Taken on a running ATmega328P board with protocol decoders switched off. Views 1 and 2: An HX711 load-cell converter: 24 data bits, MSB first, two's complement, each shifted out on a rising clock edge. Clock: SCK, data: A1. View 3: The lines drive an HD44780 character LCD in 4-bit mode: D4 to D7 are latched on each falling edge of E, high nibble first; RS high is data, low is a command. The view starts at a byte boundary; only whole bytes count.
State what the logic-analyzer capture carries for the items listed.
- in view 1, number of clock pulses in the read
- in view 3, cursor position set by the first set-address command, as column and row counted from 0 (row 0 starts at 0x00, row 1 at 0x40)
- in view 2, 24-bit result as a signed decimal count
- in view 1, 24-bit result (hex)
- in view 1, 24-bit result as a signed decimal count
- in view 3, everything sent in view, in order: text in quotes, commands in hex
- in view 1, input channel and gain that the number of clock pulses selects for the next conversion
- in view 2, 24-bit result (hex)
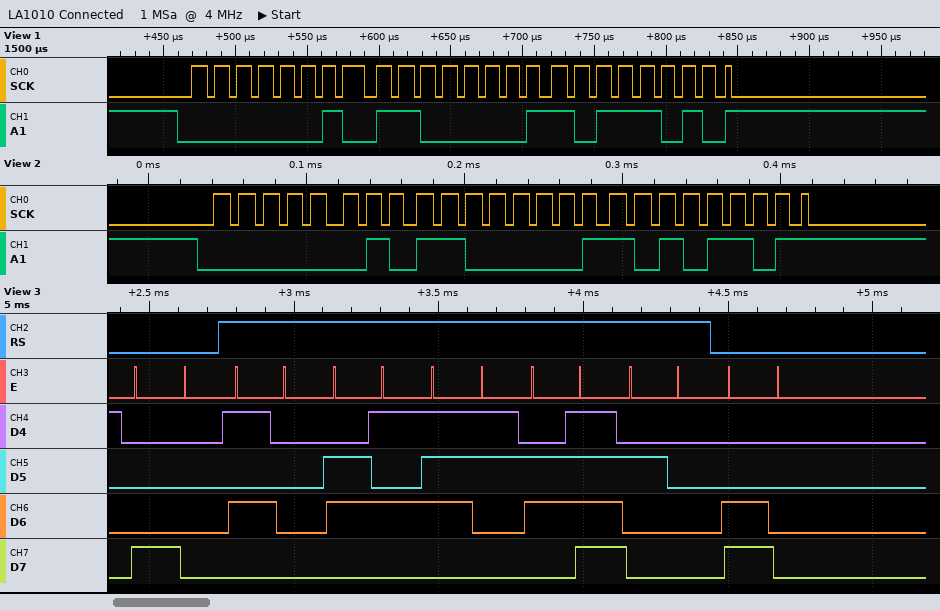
25
column 0, row 0
180653
0x02C1BA
180666
0x80 "Peso " 0xC0
channel A, gain 128
0x02C1AD
